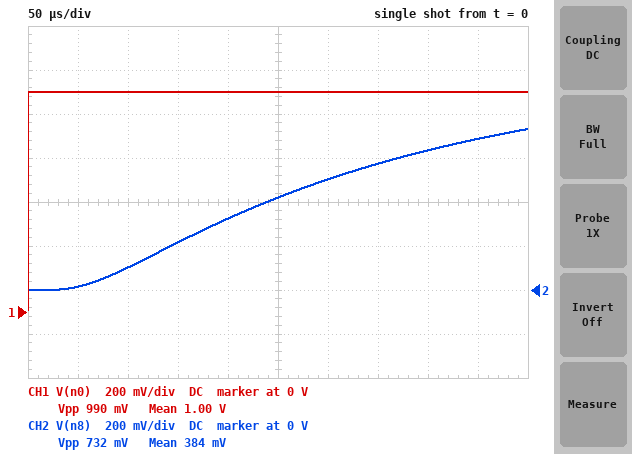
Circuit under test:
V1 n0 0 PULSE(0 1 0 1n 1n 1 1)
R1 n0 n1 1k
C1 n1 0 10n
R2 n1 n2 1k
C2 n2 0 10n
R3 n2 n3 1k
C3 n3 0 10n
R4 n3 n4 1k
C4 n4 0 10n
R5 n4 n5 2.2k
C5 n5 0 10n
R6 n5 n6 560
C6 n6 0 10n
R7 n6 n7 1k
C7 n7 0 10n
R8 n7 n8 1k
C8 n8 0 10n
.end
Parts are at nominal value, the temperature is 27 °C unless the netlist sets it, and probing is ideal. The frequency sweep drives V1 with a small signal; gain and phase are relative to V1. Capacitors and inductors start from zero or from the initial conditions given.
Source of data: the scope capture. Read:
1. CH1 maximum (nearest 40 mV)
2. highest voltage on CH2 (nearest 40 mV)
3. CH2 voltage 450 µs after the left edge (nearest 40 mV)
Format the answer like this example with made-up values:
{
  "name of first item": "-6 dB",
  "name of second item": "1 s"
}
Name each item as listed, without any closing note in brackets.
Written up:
{
  "CH1 maximum": "1.00 V",
  "highest voltage on CH2": "720 mV",
  "CH2 voltage 450 µs after the left edge": "680 mV"
}
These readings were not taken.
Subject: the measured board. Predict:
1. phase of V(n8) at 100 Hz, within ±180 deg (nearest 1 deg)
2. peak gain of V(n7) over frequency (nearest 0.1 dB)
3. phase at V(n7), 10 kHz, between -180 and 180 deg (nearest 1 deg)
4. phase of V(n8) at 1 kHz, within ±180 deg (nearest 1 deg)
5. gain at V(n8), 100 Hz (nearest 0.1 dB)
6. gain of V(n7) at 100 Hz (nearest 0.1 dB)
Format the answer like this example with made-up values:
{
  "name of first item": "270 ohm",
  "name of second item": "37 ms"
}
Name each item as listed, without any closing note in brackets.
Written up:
{
  "phase of V(n8) at 100 Hz, within ±180 deg": "-14 deg",
  "peak gain of V(n7) over frequency": "0 dB",
  "phase at V(n7), 10 kHz, between -180 and 180 deg": "126 deg",
  "phase of V(n8) at 1 kHz, within ±180 deg": "-89 deg",
  "gain at V(n8), 100 Hz": "-0.2 dB",
  "gain of V(n7) at 100 Hz": "-0.2 dB"
}
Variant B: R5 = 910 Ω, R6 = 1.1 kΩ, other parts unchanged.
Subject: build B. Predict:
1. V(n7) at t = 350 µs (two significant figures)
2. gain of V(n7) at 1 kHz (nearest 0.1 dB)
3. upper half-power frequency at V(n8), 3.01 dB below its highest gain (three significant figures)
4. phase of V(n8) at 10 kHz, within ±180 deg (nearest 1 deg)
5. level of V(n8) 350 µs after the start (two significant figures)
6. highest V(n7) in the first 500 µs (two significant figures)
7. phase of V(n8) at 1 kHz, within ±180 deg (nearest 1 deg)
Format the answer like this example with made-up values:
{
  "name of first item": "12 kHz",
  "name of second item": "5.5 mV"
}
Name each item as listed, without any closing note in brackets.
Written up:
{
  "V(n7) at t = 350 µs": "630 mV",
  "gain of V(n7) at 1 kHz": "-6.6 dB",
  "upper half-power frequency at V(n8), 3.01 dB below its highest gain": "535 Hz",
  "phase of V(n8) at 10 kHz, within ±180 deg": "99 deg",
  "level of V(n8) 350 µs after the start": "620 mV",
  "highest V(n7) in the first 500 µs": "780 mV",
  "phase of V(n8) at 1 kHz, within ±180 deg": "-85 deg"
}
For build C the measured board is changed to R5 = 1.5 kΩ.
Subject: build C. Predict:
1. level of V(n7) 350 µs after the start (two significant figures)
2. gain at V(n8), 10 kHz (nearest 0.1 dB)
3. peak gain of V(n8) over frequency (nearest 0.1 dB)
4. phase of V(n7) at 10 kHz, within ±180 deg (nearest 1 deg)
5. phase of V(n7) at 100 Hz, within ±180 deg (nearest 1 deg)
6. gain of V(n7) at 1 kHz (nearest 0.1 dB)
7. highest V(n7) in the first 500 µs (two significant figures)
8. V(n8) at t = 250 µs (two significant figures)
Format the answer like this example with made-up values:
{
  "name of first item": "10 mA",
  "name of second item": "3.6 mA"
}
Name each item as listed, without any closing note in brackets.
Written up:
{
  "level of V(n7) 350 µs after the start": "620 mV",
  "gain at V(n8), 10 kHz": "-36.5 dB",
  "peak gain of V(n8) over frequency": "0 dB",
  "phase of V(n7) at 10 kHz, within ±180 deg": "132 deg",
  "phase of V(n7) at 100 Hz, within ±180 deg": "-13 deg",
  "gain of V(n7) at 1 kHz": "-6.8 dB",
  "highest V(n7) in the first 500 µs": "770 mV",
  "V(n8) at t = 250 µs": "450 mV"
}
